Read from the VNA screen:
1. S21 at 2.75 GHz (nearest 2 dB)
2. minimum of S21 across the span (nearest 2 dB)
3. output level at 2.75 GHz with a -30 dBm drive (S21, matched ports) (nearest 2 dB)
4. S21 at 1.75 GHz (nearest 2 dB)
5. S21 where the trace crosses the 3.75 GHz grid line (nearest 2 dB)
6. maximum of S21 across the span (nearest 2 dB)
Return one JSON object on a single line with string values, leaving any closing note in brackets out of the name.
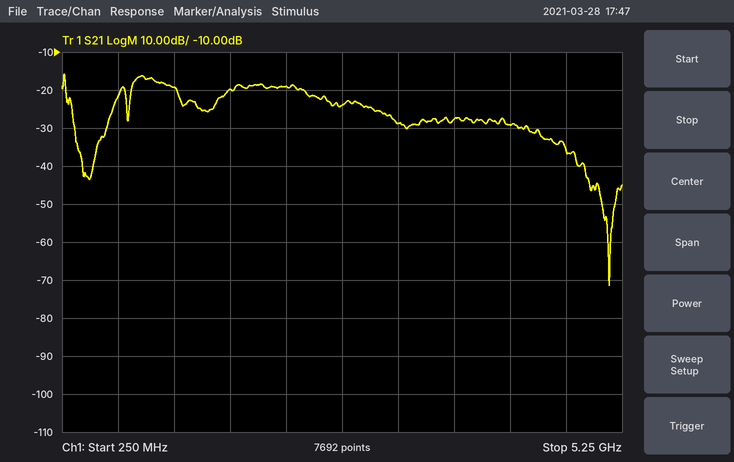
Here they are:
{"S21 at 2.75 GHz": "-24 dB", "minimum of S21 across the span": "-72 dB", "output level at 2.75 GHz with a -30 dBm drive (S21, matched ports)": "-54 dBm", "S21 at 1.75 GHz": "-20 dB", "S21 where the trace crosses the 3.75 GHz grid line": "-28 dB", "maximum of S21 across the span": "-16 dB"}
